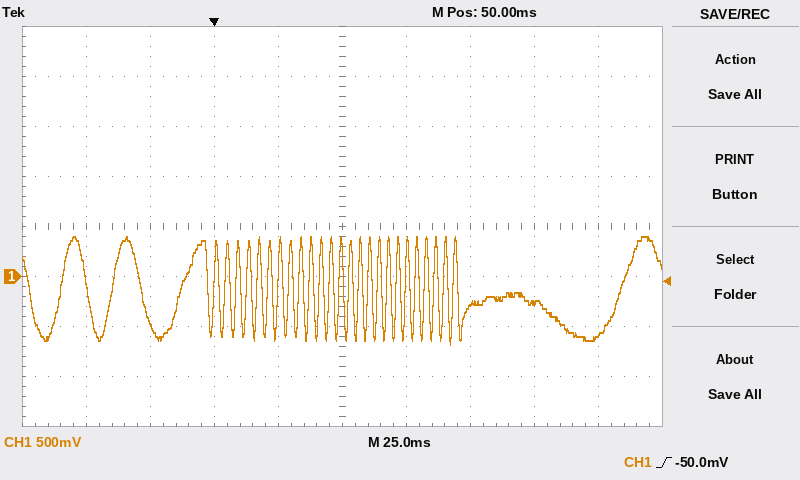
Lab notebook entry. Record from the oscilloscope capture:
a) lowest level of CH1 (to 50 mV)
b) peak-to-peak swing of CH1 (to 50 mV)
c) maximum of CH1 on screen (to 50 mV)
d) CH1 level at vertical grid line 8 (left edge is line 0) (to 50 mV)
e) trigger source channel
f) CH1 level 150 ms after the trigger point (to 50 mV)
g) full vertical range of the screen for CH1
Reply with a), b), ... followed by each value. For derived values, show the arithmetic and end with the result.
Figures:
a) -700 mV
b) 400 mV − (-700 mV) = 1.10 V
c) 400 mV
d) -250 mV
e) CH1
f) -600 mV
g) 4 V
